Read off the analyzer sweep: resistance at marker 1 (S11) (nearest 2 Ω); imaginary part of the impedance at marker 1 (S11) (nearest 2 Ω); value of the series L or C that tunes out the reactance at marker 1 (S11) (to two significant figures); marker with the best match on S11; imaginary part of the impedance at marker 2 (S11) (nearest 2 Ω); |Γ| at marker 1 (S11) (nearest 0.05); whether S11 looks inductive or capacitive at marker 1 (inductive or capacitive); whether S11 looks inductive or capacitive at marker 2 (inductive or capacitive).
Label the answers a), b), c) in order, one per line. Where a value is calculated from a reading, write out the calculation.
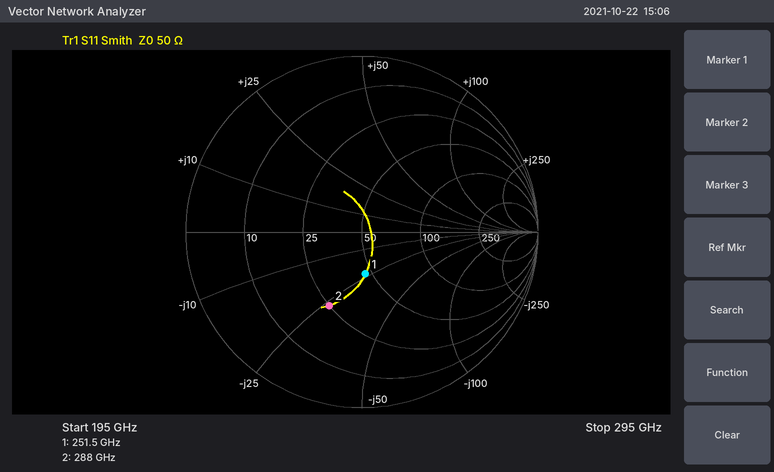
a) 46 Ω
b) -24 Ω
c) L = 24 Ω/(2π × 251.5 GHz) ≈ 15 pH
d) marker 1
e) -26 Ω
f) 0.25
g) capacitive
h) capacitive
